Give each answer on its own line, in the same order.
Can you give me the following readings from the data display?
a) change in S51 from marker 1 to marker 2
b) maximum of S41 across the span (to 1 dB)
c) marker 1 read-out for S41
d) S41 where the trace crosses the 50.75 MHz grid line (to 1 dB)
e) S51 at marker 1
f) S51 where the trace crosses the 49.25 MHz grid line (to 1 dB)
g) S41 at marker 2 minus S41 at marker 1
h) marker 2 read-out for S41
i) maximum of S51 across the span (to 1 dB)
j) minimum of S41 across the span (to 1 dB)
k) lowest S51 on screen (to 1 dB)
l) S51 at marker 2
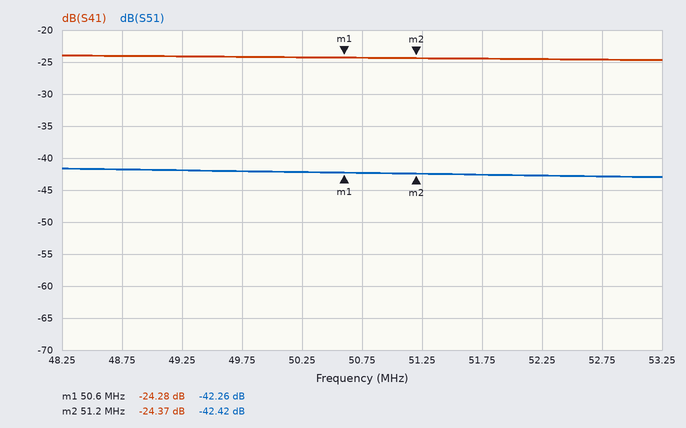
-0.16 dB
-24 dB
-24.28 dB
-24 dB
-42.26 dB
-42 dB
-0.09 dB
-24.37 dB
-42 dB
-25 dB
-43 dB
-42.42 dB
